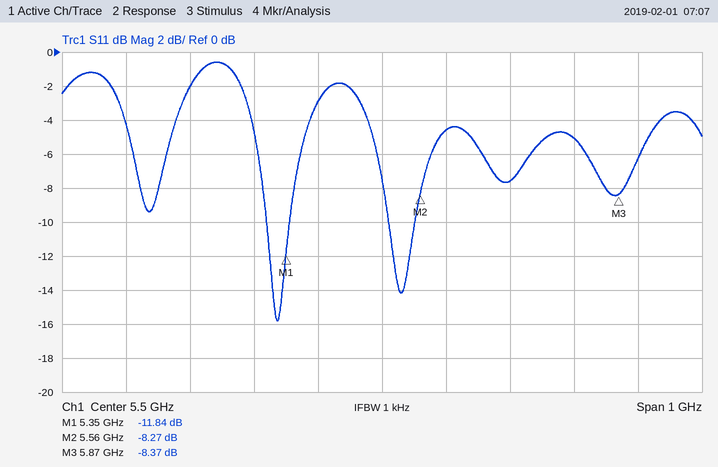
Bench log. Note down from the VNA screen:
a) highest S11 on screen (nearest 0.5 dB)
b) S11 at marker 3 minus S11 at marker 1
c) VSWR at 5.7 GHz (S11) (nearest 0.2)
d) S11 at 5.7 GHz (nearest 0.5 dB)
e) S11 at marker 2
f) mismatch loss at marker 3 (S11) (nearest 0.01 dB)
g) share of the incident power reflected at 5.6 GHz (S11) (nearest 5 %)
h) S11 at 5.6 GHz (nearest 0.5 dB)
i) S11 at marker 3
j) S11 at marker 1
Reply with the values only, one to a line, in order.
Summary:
-0.5 dB
3.47 dB
2.4
-7.5 dB
-8.27 dB
0.68 dB
35 %
-4.5 dB
-8.37 dB
-11.84 dB
